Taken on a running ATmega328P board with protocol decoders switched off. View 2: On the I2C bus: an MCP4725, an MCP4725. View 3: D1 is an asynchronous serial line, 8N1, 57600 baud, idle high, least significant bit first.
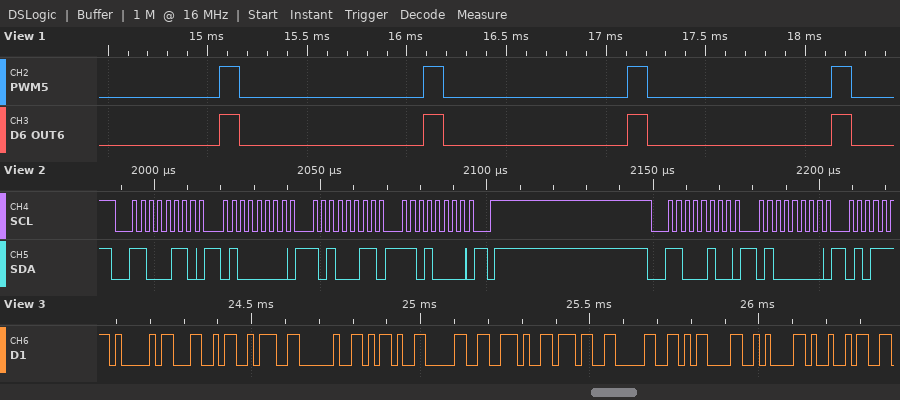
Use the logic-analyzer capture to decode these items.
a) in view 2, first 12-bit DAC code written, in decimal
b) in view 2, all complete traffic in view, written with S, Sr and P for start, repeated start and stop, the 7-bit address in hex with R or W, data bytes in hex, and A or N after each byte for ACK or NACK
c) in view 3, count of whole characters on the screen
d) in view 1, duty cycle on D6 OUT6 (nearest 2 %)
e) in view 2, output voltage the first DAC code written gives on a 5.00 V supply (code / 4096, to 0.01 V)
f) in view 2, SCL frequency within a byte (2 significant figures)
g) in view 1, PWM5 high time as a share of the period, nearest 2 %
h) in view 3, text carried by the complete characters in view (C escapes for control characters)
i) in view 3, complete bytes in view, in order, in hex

2621
S 63W A 40 A A3 A D0 A P S 62W A 40 A
12
10 %
3.20 V
400 kHz
10 %
"AL: -0.70\r\nI"
41 4C 3A 20 2D 30 2E 37 30 0D 0A 49
